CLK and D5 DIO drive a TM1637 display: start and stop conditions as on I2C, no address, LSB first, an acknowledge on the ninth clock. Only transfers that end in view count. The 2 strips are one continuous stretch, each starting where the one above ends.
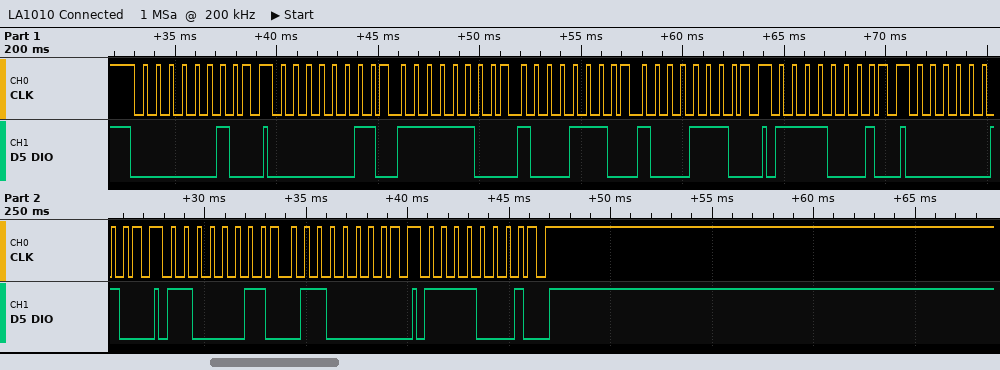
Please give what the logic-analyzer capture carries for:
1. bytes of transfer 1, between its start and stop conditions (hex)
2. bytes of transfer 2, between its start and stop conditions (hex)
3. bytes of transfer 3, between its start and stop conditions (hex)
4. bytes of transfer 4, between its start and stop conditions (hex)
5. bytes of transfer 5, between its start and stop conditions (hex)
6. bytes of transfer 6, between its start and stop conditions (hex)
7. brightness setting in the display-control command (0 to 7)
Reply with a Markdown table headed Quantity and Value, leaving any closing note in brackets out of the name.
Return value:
| Quantity | Value |
|---|---|
| bytes of transfer 1, between its start and stop conditions | 40 |
| bytes of transfer 2, between its start and stop conditions | C0 3F 71 71 |
| bytes of transfer 3, between its start and stop conditions | 8F |
| bytes of transfer 4, between its start and stop conditions | 40 |
| bytes of transfer 5, between its start and stop conditions | C3 06 |
| bytes of transfer 6, between its start and stop conditions | 8F |
| brightness setting in the display-control command | 7 |
